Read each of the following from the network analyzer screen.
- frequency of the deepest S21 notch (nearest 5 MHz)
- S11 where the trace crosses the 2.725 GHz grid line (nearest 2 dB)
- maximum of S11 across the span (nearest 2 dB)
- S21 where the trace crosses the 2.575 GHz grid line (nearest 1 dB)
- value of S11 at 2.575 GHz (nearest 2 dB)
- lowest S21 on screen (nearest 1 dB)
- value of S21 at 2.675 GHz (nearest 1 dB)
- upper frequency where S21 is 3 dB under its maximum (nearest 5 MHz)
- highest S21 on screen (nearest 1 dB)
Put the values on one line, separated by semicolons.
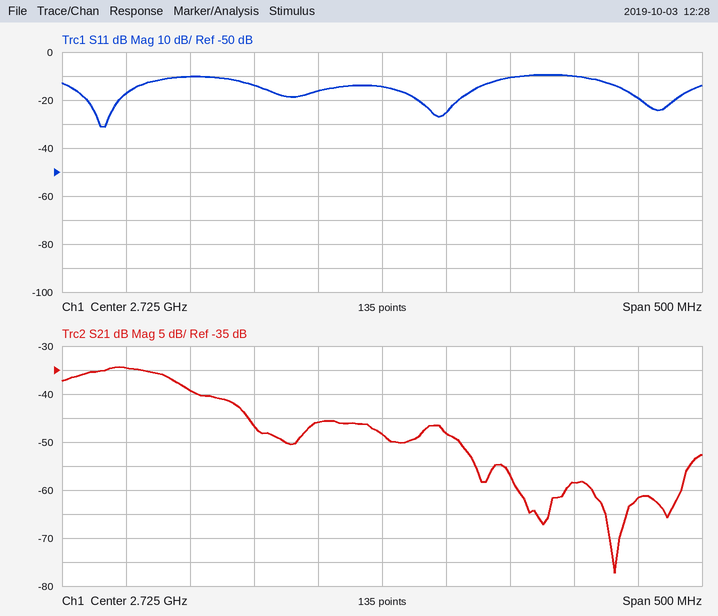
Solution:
2.905 GHz; -14 dB; -10 dB; -39 dB; -10 dB; -77 dB; -46 dB; 2.565 GHz; -34 dB
